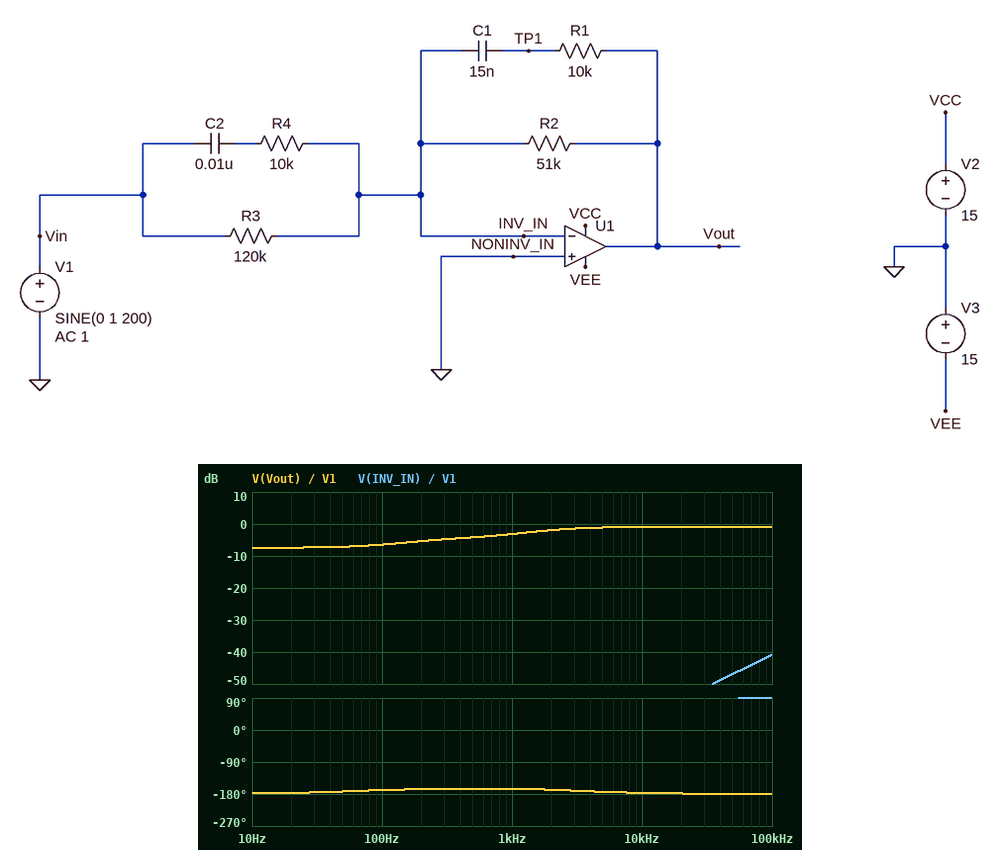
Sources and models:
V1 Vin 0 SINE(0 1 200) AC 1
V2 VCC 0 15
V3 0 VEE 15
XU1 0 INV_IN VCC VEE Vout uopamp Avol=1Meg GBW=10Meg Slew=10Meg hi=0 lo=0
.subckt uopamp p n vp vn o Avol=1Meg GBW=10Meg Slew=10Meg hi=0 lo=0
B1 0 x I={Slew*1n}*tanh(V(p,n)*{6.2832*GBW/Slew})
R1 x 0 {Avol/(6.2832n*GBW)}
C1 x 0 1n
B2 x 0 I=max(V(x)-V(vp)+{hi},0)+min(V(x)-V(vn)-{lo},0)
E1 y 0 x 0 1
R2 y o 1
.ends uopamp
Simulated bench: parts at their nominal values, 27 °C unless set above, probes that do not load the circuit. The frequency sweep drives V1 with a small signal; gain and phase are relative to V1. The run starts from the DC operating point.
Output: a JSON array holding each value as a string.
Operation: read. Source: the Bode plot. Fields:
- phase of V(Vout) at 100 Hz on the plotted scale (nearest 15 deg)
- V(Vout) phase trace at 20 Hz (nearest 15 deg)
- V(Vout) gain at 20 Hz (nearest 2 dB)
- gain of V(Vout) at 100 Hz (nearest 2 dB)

["-165 deg", "-180 deg", "-8 dB", "-6 dB"]
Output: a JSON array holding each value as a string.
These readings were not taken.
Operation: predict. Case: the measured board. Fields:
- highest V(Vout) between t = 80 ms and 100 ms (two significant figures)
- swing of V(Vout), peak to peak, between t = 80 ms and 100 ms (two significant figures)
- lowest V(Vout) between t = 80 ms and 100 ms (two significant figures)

["540 mV", "1.1 V", "-540 mV"]
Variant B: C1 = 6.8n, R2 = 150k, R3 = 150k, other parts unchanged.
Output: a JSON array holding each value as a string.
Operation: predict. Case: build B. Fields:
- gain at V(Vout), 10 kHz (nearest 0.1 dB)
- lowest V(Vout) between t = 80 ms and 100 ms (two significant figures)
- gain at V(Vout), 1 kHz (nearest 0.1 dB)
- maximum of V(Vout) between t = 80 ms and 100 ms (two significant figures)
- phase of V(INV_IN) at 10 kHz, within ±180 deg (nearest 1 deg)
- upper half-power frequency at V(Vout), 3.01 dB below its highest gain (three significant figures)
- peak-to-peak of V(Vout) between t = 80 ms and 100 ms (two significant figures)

["0.1 dB", "-1.3 V", "2.6 dB", "1.3 V", "86 deg", "600 kHz", "2.6 V"]
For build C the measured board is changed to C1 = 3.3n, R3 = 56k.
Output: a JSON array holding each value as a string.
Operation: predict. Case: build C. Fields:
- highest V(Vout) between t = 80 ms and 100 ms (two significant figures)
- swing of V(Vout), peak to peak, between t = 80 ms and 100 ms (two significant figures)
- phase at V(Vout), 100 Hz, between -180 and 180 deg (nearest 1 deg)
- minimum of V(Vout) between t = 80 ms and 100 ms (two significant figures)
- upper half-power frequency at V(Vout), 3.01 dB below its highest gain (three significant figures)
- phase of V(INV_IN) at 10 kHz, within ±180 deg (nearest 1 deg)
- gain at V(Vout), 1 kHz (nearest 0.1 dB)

["1.1 V", "2.3 V", "-167 deg", "-1.1 V", "3.56 kHz", "76 deg", "6.4 dB"]
